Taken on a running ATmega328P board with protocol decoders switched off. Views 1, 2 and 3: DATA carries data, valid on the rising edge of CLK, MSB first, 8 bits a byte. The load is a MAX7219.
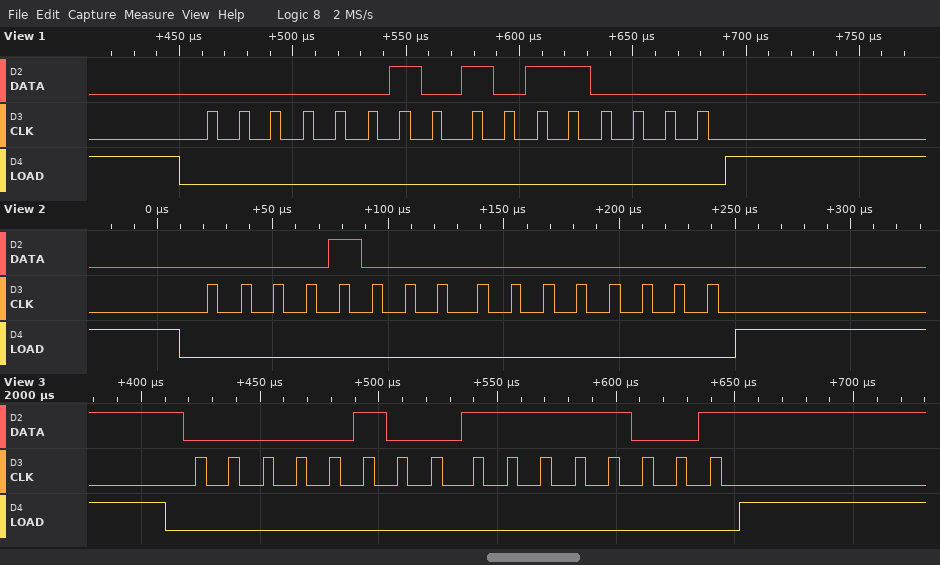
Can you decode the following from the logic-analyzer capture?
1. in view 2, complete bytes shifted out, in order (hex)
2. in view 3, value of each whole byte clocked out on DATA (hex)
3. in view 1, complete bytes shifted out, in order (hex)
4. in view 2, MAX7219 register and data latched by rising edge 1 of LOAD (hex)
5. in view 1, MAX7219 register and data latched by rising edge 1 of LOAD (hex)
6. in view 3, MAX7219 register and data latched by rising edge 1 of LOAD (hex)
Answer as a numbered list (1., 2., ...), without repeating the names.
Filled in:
1. 08 00
2. 04 F9
3. 0x02 0xB0
4. register 0x8, data 0x00
5. register 0x2, data 0xB0
6. register 0x4, data 0xF9
